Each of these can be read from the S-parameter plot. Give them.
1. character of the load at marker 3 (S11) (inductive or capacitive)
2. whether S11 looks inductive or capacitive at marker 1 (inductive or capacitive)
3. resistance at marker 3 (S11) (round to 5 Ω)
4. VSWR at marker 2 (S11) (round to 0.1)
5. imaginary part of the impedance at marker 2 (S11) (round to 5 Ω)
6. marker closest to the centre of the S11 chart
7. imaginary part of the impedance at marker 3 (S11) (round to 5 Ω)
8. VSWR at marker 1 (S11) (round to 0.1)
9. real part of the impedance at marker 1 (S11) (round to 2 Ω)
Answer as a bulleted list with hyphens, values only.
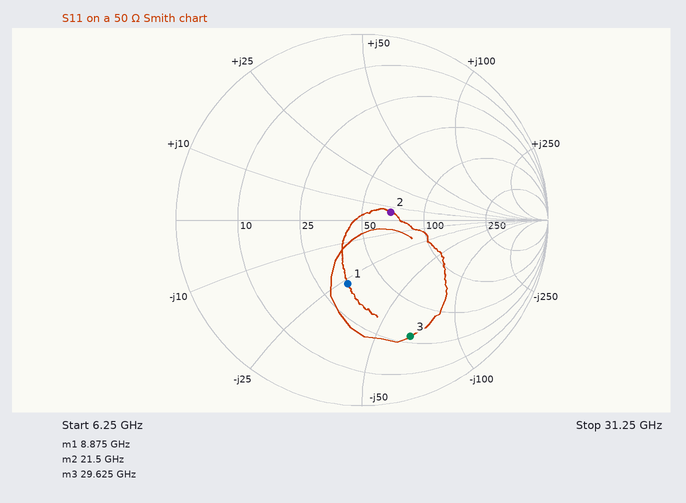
- capacitive
- capacitive
- 30 Ω
- 1.4
- +5 Ω
- marker 2
- -65 Ω
- 2.1
- 34 Ω
